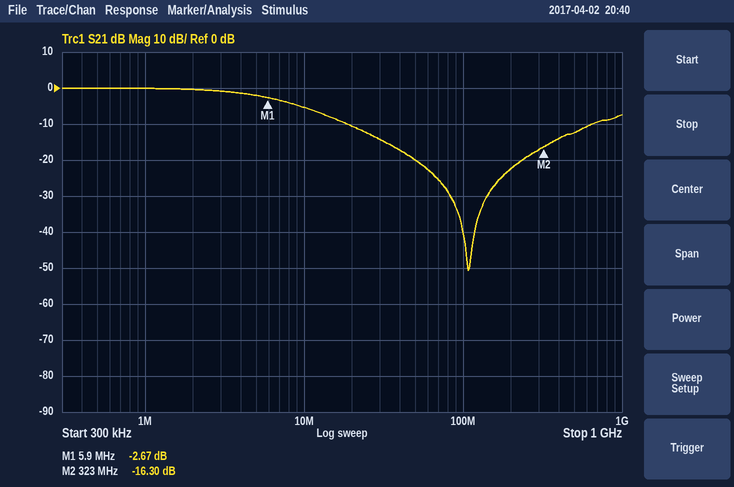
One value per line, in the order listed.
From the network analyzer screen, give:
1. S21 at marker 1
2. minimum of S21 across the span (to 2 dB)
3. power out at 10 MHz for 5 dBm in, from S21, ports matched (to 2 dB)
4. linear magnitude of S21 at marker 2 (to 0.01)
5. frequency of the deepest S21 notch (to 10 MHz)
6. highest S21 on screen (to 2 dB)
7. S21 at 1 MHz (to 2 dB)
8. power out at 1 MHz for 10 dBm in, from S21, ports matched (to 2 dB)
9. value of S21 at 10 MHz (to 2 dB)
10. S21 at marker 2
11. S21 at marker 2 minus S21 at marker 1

-2.67 dB
-50 dB
0 dBm
0.15
110 MHz
0 dB
0 dB
10 dBm
-6 dB
-16.30 dB
-13.63 dB
